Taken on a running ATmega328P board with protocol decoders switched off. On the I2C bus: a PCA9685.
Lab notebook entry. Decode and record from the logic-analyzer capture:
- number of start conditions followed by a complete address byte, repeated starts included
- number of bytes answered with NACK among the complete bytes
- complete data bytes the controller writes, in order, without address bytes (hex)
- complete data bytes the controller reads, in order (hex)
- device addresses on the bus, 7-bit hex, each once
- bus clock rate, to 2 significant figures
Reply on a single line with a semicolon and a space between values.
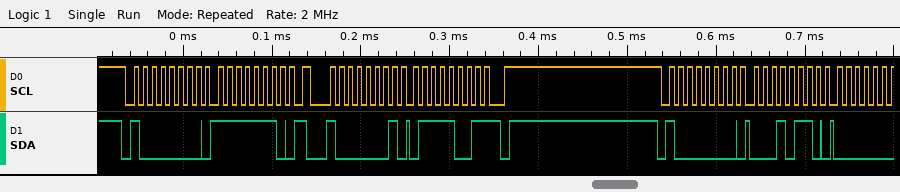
3; 1; FE 16; 79; 0x40; 100 kHz
